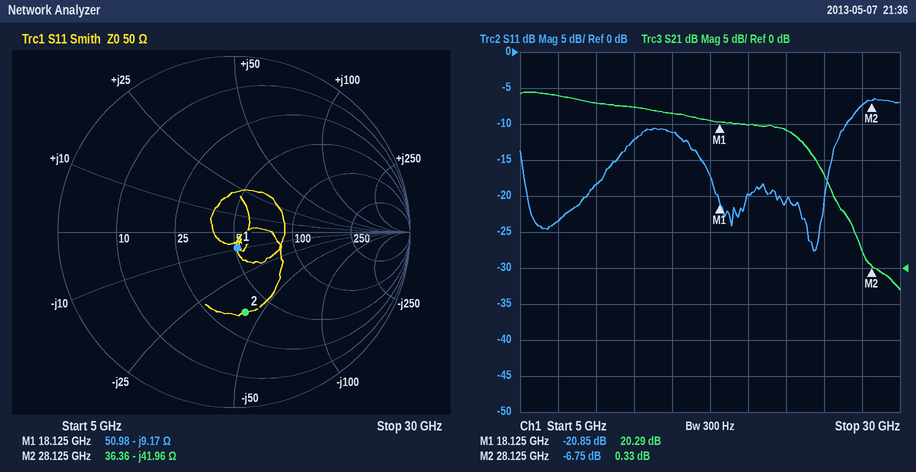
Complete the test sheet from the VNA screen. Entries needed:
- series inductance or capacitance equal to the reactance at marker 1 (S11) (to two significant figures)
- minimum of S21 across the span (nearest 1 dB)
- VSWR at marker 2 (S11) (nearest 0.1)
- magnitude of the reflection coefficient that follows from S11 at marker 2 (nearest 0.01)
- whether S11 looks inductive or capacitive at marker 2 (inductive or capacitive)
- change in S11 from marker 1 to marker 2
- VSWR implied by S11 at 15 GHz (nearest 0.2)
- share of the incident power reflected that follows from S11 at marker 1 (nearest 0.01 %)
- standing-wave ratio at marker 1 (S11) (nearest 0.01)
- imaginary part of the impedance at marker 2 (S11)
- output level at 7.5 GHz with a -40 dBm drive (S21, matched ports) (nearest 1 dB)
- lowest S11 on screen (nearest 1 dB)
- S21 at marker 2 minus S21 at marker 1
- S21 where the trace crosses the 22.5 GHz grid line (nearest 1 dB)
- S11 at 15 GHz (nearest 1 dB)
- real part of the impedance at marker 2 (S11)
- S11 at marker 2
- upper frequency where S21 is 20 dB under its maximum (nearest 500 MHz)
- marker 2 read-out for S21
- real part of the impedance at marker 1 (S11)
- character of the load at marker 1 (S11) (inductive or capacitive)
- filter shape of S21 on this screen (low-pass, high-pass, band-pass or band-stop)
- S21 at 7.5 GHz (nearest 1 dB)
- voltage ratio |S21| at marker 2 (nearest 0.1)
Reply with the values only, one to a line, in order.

960 fF
-3 dB
2.7
0.46
capacitive
14.10 dB
1.8
0.82 %
1.20
-41.96 Ω
-16 dBm
-28 dB
-19.96 dB
19 dB
-11 dB
36.36 Ω
-6.75 dB
27.0 GHz
0.33 dB
50.98 Ω
capacitive
low-pass
24 dB
1.0
